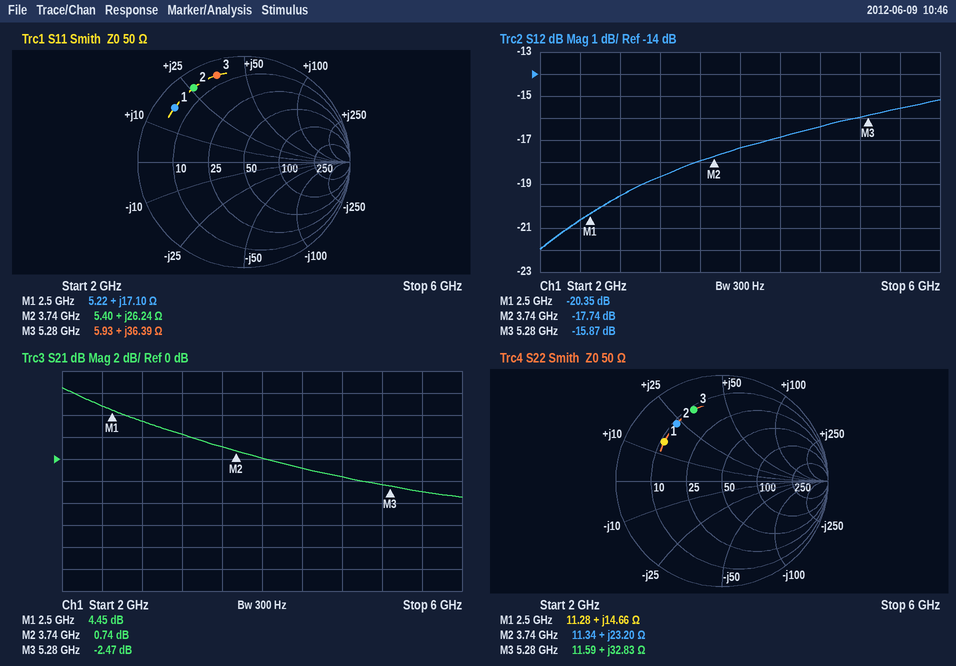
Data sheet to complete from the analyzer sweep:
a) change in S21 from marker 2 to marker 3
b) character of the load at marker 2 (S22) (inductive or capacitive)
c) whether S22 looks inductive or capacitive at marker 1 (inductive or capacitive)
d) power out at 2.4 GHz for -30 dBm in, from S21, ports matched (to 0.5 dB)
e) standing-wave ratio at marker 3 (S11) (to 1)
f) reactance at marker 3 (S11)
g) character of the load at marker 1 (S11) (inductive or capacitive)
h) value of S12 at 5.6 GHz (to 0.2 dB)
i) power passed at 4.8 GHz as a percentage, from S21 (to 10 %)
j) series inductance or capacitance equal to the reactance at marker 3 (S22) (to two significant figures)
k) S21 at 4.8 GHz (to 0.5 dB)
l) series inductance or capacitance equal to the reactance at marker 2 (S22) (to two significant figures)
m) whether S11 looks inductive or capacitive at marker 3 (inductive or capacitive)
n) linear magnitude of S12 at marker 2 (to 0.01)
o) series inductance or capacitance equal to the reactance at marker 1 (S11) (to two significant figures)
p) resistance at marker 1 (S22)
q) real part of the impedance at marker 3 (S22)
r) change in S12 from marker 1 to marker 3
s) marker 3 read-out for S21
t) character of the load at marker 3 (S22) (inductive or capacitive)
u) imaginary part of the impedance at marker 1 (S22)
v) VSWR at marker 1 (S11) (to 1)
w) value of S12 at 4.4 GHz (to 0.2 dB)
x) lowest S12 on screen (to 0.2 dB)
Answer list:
-3.21 dB
inductive
inductive
-25.0 dBm
13
+36.39 Ω
inductive
-15.6 dB
70 %
990 pH
-1.5 dB
990 pH
inductive
0.13
1.1 nH
11.28 Ω
11.59 Ω
4.48 dB
-2.47 dB
inductive
+14.66 Ω
11
-16.8 dB
-22.0 dB
